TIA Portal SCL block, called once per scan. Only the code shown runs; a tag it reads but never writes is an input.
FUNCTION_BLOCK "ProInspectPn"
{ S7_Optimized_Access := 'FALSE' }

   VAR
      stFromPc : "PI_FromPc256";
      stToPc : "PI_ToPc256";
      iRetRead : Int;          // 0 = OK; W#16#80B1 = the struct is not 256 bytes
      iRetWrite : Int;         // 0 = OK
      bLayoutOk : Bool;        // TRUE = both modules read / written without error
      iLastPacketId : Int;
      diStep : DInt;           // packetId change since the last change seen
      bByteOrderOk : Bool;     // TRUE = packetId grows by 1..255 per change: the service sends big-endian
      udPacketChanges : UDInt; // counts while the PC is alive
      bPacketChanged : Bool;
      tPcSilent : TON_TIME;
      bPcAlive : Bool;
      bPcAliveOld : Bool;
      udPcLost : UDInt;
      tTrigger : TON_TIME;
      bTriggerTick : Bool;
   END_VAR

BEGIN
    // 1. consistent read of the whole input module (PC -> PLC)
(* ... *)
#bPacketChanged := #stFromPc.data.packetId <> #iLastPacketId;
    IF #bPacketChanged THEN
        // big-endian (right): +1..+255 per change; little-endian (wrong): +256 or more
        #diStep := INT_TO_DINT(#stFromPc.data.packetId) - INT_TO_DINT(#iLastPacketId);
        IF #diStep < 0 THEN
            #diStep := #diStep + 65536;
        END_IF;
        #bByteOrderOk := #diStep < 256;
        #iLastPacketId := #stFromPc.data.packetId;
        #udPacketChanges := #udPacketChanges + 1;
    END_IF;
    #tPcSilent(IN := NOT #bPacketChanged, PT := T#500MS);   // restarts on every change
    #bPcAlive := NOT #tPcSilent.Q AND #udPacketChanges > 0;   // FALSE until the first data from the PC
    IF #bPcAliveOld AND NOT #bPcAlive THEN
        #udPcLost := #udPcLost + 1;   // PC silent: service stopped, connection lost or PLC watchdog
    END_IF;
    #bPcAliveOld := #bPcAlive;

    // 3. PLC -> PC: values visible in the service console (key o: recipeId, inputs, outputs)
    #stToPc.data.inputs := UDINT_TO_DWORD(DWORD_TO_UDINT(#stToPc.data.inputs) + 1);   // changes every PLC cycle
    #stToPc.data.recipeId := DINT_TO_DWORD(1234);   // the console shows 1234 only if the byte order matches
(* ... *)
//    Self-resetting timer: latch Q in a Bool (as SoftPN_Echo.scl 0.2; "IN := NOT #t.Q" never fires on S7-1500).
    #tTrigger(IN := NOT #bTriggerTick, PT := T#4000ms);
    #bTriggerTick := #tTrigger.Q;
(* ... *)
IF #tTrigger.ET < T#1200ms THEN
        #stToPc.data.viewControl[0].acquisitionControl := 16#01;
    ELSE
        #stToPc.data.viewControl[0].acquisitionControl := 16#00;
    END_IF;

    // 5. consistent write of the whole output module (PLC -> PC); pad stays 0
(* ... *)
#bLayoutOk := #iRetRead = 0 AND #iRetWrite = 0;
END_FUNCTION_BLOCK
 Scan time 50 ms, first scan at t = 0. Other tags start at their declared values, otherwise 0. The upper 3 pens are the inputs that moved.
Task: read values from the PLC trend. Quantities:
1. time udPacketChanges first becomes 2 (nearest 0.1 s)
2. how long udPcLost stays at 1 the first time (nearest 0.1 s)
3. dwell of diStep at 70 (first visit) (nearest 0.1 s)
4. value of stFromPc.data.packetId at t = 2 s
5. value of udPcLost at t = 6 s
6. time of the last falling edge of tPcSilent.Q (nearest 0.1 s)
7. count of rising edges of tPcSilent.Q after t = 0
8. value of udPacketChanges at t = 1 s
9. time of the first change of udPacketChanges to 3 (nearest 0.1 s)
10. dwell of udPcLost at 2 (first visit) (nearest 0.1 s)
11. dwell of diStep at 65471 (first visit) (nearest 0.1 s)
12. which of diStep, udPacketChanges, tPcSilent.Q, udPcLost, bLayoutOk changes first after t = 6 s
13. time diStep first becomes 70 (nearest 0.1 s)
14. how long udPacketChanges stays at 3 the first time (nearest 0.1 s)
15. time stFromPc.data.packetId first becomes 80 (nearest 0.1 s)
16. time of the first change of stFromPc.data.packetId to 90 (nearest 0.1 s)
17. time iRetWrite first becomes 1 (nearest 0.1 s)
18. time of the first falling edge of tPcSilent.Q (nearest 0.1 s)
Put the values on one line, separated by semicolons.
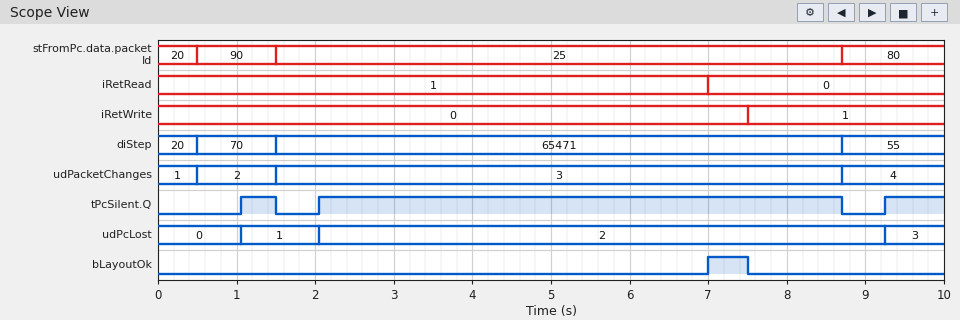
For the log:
0.5 s; 1.0 s; 1.0 s; 25; 2; 8.7 s; 3; 2; 1.5 s; 7.2 s; 7.2 s; bLayoutOk; 0.5 s; 7.2 s; 8.7 s; 0.5 s; 7.5 s; 1.5 s
